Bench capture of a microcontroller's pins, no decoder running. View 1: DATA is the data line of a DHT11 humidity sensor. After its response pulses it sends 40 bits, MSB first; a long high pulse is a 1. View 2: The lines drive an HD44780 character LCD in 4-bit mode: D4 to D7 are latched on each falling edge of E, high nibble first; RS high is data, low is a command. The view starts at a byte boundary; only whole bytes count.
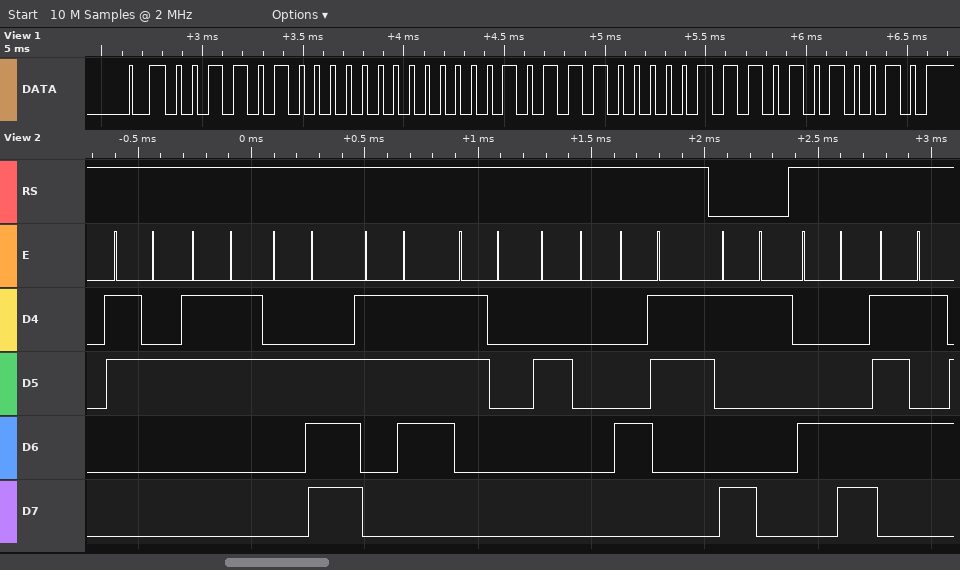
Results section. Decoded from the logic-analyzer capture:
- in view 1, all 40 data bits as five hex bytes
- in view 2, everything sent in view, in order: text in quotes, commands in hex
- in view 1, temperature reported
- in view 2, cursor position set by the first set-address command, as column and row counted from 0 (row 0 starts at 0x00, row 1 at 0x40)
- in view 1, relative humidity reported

34 00 17 07 52
"23.70 C" 0x91 "Lu"
23.7 °C
column 17, row 0
52 %
